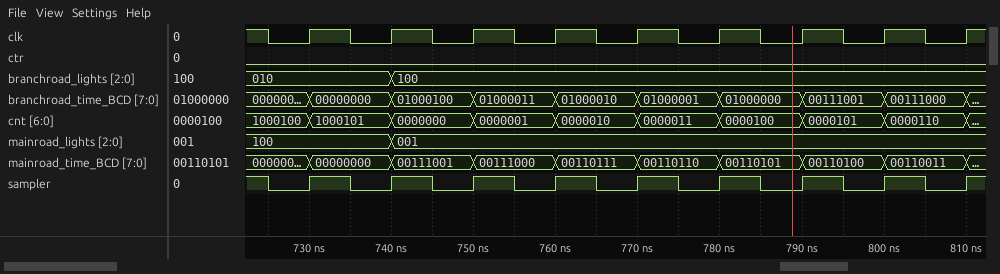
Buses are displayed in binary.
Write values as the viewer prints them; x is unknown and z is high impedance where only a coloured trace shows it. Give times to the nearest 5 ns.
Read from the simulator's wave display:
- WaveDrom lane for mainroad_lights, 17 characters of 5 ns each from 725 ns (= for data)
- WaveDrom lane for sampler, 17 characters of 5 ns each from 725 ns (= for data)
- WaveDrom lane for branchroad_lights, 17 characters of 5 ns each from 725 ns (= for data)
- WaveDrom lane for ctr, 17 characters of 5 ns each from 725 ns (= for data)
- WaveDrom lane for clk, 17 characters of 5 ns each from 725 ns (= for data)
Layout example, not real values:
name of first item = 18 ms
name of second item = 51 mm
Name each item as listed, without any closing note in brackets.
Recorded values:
WaveDrom lane for mainroad_lights, 17 characters of 5 ns each from 725 ns = {name: 'mainroad_lights', wave: '=..=.............', data: '100 001'}
WaveDrom lane for sampler, 17 characters of 5 ns each from 725 ns = {name: 'sampler', wave: '01010101010101010'}
WaveDrom lane for branchroad_lights, 17 characters of 5 ns each from 725 ns = {name: 'branchroad_lights', wave: '=..=.............', data: '010 100'}
WaveDrom lane for ctr, 17 characters of 5 ns each from 725 ns = {name: 'ctr', wave: '0................'}
WaveDrom lane for clk, 17 characters of 5 ns each from 725 ns = {name: 'clk', wave: '01010101010101010'}
